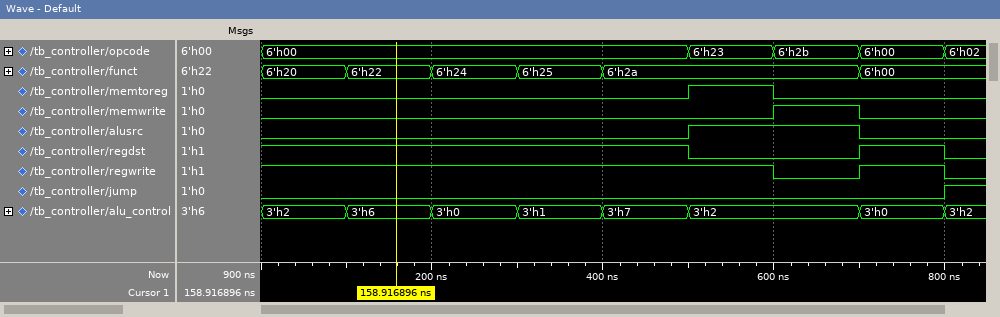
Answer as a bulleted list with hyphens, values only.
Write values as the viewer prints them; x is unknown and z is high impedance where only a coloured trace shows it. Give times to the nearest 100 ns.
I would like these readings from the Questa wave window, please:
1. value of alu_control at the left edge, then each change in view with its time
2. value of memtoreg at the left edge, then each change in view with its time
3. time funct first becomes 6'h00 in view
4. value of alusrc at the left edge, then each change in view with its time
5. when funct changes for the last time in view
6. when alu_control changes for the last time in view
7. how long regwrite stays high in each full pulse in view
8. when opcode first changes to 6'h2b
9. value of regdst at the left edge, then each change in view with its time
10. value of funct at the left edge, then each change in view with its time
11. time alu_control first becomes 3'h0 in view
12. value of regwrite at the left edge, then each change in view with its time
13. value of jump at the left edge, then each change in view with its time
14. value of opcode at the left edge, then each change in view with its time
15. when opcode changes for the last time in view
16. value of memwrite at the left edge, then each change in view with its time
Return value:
- 3'h2, 3'h6 at 100 ns, 3'h0 at 200 ns, 3'h1 at 300 ns, 3'h7 at 400 ns, 3'h2 at 500 ns, 3'h0 at 700 ns, 3'h2 at 800 ns
- 0, 1 at 500 ns, 0 at 600 ns
- 700 ns
- 0, 1 at 500 ns, 0 at 700 ns
- 700 ns
- 800 ns
- 100 ns
- 600 ns
- 1, 0 at 500 ns, 1 at 700 ns, 0 at 800 ns
- 6'h20, 6'h22 at 100 ns, 6'h24 at 200 ns, 6'h25 at 300 ns, 6'h2a at 400 ns, 6'h00 at 700 ns
- 200 ns
- 1, 0 at 600 ns, 1 at 700 ns, 0 at 800 ns
- 0, 1 at 800 ns
- 6'h00, 6'h23 at 500 ns, 6'h2b at 600 ns, 6'h00 at 700 ns, 6'h02 at 800 ns
- 800 ns
- 0, 1 at 600 ns, 0 at 700 ns
